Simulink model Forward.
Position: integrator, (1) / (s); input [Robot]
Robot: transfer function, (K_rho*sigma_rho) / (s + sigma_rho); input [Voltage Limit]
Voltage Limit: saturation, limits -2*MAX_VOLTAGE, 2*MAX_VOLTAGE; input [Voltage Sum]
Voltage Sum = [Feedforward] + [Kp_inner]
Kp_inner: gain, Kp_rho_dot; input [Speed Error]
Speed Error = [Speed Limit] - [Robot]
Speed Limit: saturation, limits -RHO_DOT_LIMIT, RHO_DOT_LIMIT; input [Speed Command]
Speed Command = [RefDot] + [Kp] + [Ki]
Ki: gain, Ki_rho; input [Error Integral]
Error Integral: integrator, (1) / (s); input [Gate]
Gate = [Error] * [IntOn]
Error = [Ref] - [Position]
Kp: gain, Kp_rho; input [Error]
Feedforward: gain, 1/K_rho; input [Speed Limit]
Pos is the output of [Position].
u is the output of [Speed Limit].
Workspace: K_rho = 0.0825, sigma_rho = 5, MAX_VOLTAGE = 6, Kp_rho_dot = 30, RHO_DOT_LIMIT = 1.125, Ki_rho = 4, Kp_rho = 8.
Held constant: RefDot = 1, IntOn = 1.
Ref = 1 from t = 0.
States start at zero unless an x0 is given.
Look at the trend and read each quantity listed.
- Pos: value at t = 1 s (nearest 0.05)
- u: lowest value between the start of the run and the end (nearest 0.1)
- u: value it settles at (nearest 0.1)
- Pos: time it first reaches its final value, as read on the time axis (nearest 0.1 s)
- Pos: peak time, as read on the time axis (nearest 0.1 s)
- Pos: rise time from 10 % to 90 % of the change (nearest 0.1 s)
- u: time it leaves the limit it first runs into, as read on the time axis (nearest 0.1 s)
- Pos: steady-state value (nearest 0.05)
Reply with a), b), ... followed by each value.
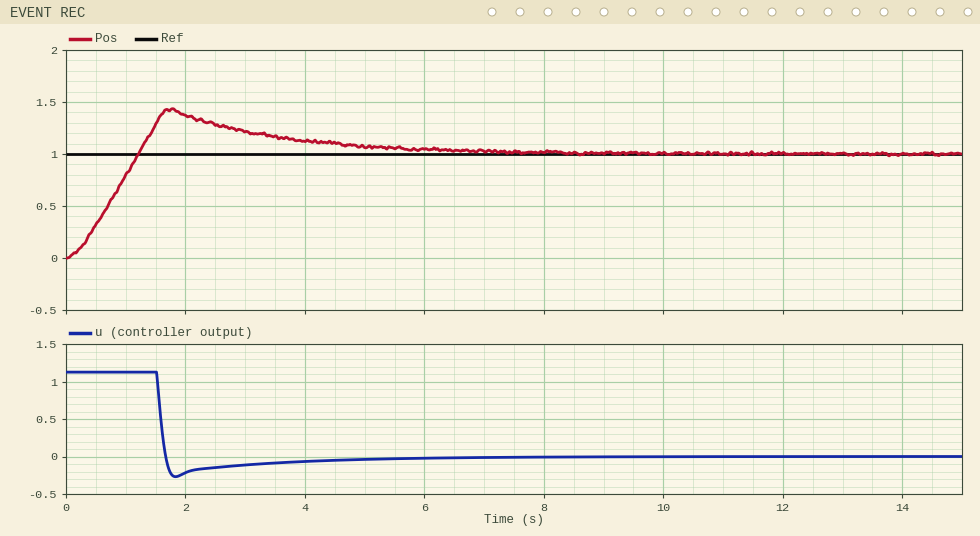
a) 0.80
b) -0.3
c) 0.0
d) 1.2 s
e) 1.7 s
f) 0.9 s
g) 1.5 s
h) 1.00
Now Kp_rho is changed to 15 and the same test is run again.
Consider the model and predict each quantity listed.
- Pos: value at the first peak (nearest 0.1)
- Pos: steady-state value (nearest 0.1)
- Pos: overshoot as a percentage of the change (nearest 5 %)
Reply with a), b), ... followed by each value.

a) 1.3
b) 1.0
c) 25 %
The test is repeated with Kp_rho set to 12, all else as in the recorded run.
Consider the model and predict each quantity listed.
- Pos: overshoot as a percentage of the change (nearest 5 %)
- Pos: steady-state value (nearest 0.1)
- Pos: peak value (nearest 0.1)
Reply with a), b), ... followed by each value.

a) 30 %
b) 1.0
c) 1.3
